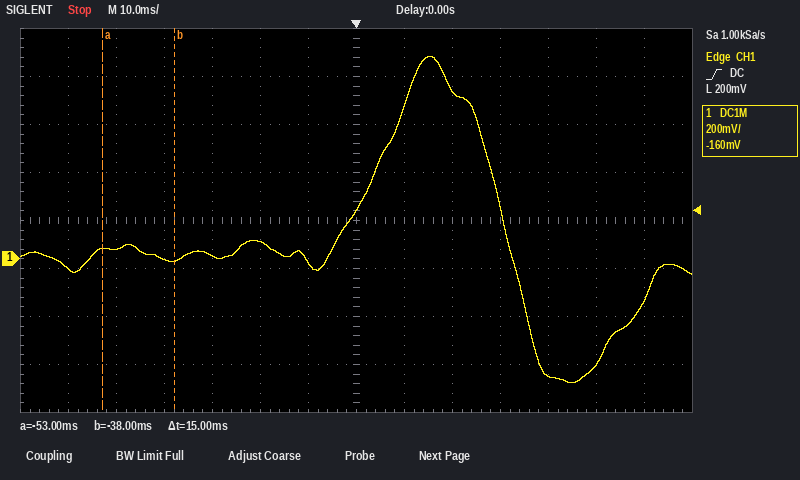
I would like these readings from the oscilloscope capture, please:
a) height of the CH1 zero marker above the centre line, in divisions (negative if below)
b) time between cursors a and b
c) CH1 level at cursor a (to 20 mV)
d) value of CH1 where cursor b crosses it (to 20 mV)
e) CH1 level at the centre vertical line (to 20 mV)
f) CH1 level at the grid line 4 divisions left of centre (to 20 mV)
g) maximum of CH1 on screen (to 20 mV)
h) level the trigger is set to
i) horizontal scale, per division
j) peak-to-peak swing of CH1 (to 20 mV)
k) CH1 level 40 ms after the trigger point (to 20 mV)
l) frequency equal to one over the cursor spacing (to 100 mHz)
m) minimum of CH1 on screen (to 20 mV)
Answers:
-0.8 div
15 ms
40 mV
0 mV
200 mV
0 mV
840 mV
200 mV
10 ms
1.36 V
-480 mV
66.7 Hz
-520 mV
